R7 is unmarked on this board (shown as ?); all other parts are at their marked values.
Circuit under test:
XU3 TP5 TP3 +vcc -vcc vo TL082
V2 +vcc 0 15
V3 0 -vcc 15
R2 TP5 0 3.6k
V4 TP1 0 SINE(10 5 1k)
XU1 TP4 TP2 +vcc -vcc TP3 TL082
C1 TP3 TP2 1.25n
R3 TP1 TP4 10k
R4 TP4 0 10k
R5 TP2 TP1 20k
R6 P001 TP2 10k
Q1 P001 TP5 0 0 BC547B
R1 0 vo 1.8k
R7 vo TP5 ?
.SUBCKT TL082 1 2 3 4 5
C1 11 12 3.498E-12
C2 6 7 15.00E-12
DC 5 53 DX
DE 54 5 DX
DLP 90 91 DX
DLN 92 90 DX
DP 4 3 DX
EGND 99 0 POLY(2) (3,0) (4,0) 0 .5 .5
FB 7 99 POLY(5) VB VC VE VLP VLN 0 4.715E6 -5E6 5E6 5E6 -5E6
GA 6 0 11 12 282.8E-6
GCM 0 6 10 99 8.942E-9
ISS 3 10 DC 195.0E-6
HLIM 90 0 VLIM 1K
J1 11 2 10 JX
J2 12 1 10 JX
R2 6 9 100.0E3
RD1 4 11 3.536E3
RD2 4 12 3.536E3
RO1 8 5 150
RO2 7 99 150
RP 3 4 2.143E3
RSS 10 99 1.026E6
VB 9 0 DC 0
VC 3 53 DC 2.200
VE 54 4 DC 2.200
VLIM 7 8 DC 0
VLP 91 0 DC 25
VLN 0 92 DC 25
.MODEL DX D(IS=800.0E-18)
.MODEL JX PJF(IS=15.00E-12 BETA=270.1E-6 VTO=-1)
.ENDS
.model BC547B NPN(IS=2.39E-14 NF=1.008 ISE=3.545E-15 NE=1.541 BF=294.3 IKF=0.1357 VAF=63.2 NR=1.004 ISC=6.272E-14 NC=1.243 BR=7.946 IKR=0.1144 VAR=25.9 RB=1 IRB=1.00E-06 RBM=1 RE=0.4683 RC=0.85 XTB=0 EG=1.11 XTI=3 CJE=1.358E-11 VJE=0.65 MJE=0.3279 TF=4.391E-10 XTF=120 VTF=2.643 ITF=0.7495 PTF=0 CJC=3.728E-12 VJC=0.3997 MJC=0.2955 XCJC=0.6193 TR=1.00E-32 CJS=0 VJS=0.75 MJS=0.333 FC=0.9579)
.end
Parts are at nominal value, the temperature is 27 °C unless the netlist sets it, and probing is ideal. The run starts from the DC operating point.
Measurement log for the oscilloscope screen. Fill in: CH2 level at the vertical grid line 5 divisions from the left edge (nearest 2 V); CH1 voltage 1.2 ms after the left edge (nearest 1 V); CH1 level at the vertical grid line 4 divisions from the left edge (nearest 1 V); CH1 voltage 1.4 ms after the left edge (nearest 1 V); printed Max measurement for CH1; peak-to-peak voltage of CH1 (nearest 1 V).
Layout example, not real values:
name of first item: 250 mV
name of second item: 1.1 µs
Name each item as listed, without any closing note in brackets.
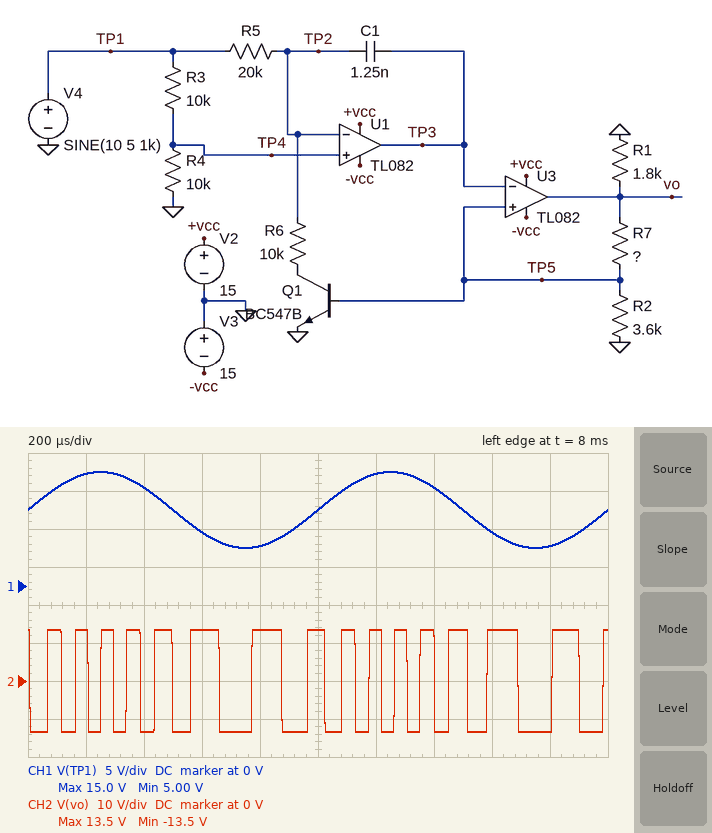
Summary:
CH2 level at the vertical grid line 5 divisions from the left edge: 14 V
CH1 voltage 1.2 ms after the left edge: 15 V
CH1 level at the vertical grid line 4 divisions from the left edge: 5 V
CH1 voltage 1.4 ms after the left edge: 13 V
printed Max measurement for CH1: 15.0 V
peak-to-peak voltage of CH1: 10 V
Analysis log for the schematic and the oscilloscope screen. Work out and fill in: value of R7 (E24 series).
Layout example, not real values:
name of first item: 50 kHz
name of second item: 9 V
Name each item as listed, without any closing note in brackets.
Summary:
value of R7: 1 kΩ
